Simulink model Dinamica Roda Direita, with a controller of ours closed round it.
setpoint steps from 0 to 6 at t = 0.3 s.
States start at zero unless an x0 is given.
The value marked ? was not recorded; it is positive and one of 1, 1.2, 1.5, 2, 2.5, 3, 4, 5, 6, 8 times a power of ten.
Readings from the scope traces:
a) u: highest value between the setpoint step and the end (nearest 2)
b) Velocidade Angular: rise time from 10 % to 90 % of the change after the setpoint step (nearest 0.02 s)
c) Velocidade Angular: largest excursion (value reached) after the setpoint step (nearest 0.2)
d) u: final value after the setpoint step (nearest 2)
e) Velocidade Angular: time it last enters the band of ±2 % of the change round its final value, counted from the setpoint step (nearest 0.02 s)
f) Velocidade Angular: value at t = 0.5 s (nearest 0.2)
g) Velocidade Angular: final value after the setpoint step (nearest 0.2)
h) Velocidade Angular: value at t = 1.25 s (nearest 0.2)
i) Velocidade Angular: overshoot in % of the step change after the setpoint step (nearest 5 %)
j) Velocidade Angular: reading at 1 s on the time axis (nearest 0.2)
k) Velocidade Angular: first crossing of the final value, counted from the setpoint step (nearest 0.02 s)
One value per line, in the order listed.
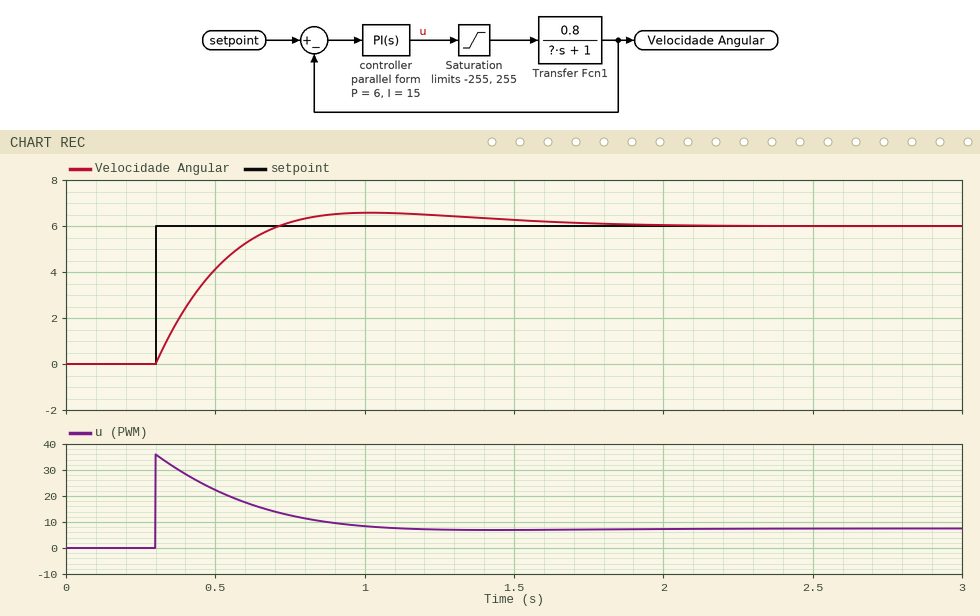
36
0.30 s
6.6
8
1.44 s
4.2
6.0
6.4
10 %
6.6
0.42 s
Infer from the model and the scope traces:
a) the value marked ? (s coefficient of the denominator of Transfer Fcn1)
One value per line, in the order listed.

1
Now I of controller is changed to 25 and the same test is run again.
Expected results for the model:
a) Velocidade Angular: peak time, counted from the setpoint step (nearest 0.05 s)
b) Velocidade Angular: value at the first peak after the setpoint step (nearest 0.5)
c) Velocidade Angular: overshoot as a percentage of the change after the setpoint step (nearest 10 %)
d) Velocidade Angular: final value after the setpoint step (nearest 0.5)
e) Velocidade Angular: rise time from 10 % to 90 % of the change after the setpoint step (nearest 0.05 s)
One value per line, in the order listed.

0.55 s
7.0
20 %
6.0
0.25 s
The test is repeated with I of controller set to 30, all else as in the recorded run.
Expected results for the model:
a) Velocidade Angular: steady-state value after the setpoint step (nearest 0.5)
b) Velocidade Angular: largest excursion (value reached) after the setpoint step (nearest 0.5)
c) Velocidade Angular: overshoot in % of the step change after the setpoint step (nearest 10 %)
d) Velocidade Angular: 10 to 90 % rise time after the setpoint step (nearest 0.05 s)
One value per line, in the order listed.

6.0
7.0
20 %
0.20 s
